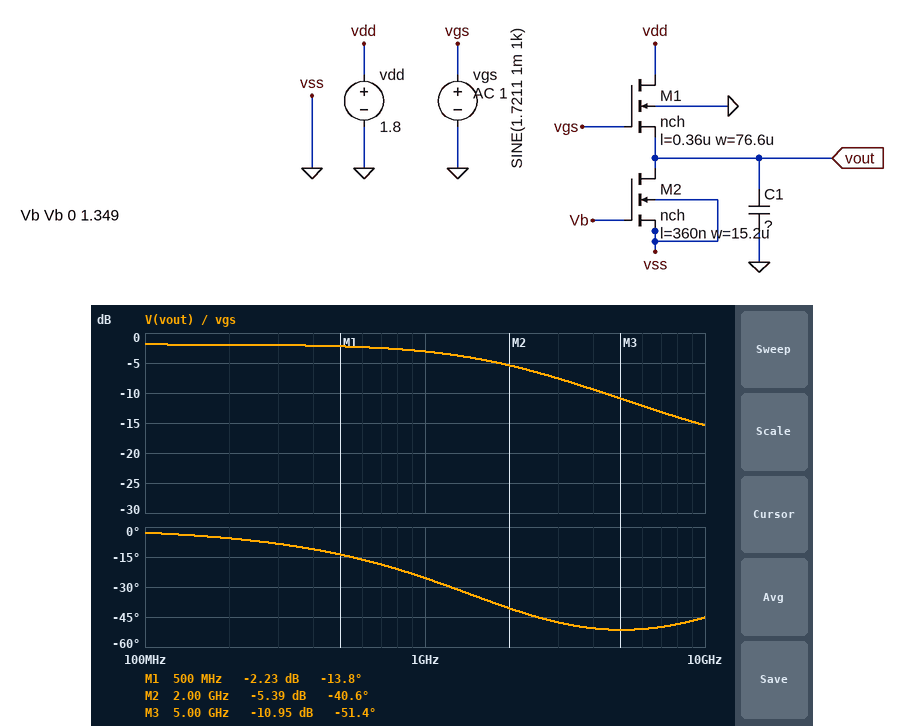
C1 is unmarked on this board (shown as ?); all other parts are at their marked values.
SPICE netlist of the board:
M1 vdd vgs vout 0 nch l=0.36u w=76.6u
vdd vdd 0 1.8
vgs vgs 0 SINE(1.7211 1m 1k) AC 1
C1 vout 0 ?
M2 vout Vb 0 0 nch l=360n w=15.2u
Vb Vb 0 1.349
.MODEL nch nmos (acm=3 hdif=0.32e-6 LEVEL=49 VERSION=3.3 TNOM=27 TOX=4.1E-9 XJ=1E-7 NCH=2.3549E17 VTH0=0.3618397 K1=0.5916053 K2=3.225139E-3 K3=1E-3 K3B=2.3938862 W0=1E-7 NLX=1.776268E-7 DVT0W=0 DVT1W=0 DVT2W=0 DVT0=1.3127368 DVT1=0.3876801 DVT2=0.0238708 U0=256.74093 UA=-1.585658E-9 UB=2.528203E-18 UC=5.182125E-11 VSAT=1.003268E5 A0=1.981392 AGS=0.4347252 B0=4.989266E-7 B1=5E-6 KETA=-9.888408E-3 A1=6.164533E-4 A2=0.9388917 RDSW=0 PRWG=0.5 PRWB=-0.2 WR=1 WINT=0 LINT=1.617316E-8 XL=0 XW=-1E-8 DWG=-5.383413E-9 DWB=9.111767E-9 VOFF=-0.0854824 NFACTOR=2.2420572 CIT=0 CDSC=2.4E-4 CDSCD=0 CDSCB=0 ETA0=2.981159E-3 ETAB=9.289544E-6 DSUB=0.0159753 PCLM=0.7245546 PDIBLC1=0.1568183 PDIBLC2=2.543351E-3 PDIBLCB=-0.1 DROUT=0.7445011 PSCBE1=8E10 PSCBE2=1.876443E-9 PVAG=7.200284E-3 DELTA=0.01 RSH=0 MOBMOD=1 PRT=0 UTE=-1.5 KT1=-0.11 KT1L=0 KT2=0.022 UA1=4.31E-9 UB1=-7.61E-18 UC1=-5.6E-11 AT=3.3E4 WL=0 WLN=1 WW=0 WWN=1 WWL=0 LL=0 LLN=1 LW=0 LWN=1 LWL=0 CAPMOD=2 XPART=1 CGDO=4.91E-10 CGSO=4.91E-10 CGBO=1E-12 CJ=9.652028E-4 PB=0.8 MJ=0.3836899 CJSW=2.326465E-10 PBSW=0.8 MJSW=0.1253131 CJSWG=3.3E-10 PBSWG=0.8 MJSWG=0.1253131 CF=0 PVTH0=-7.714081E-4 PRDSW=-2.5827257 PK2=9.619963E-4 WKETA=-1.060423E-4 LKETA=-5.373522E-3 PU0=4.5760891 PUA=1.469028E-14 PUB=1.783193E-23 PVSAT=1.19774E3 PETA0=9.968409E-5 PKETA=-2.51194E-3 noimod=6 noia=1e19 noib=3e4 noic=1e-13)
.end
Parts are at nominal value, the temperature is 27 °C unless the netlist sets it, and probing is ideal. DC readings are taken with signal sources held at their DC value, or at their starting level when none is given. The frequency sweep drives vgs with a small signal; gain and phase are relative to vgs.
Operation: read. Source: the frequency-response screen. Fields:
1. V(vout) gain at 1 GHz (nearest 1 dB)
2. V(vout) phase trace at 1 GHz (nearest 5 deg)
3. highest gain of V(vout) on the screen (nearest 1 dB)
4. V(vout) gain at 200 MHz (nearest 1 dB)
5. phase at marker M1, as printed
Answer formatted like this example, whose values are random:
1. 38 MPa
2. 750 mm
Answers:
1. -3 dB
2. -25 deg
3. -2 dB
4. -2 dB
5. -13.8 deg
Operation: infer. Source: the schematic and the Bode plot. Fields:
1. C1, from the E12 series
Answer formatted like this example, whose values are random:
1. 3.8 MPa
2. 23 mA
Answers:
1. 1.5 pF
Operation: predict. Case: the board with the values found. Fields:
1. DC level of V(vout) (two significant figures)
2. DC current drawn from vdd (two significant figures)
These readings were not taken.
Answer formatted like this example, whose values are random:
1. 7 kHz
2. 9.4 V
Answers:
1. 750 mV
2. 3.0 mA
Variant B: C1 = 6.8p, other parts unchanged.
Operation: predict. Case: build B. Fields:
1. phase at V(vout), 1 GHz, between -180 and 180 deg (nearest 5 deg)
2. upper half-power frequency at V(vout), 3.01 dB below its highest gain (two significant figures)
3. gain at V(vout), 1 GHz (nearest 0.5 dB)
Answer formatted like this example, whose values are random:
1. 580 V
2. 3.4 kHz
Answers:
1. -60 deg
2. 450 MHz
3. -9.5 dB
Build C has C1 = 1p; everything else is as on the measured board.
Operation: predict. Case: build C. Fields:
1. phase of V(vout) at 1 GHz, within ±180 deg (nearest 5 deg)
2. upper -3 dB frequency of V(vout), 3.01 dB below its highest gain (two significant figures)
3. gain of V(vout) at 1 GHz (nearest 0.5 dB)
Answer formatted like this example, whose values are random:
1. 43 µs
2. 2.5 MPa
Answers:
1. -20 deg
2. 2.5 GHz
3. -2.5 dB
